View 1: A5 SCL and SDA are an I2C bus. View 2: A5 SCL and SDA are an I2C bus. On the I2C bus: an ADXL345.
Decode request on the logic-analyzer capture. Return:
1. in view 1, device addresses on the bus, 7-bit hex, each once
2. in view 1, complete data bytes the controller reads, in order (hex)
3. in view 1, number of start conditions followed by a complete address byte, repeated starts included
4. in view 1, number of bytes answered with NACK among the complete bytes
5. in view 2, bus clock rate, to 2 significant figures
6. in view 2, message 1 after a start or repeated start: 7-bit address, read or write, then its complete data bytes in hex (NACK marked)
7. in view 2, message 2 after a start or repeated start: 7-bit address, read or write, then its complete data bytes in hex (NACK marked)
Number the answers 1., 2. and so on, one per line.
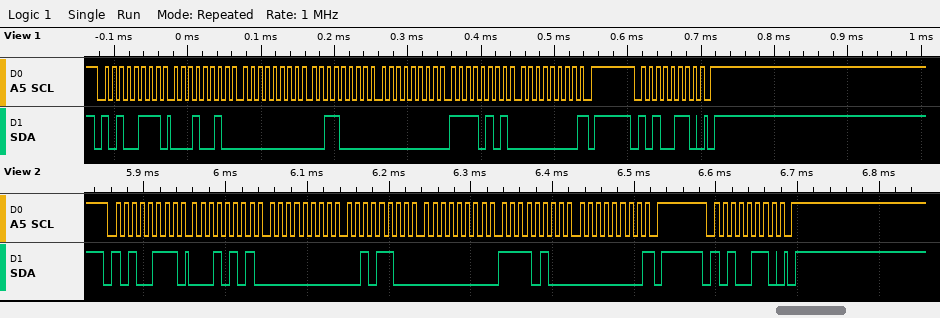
1. 0x53
2. 12 00 30 00 F5 00
3. 2
4. 1
5. 100 kHz
6. 0x53 read: 15 00 2C 00 F4 00 NACK
7. 0x53 write
